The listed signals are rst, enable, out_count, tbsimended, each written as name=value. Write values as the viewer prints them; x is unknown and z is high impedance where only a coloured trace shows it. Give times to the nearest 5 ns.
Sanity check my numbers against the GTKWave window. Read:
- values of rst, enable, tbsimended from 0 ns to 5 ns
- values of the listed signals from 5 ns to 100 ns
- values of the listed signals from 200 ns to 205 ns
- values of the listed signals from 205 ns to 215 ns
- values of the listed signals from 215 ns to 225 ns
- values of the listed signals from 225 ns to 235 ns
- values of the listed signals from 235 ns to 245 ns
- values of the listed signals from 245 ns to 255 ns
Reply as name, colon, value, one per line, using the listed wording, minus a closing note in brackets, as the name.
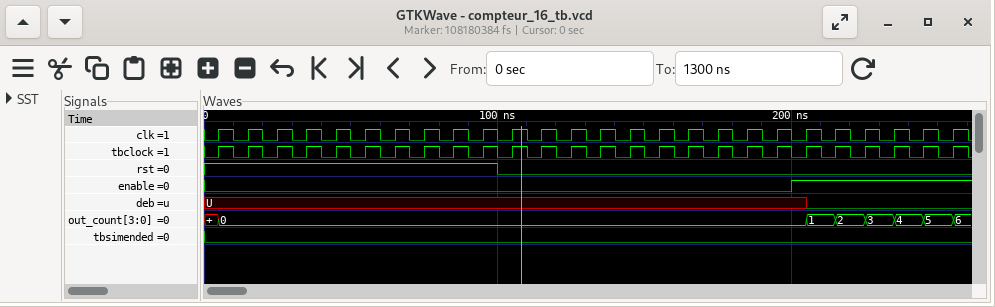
values of rst, enable, tbsimended from 0 ns to 5 ns: rst=1, enable=0, tbsimended=0
values of the listed signals from 5 ns to 100 ns: rst=1, enable=0, out_count=0, tbsimended=0
values of the listed signals from 200 ns to 205 ns: rst=0, enable=1, out_count=0, tbsimended=0
values of the listed signals from 205 ns to 215 ns: rst=0, enable=1, out_count=1, tbsimended=0
values of the listed signals from 215 ns to 225 ns: rst=0, enable=1, out_count=2, tbsimended=0
values of the listed signals from 225 ns to 235 ns: rst=0, enable=1, out_count=3, tbsimended=0
values of the listed signals from 235 ns to 245 ns: rst=0, enable=1, out_count=4, tbsimended=0
values of the listed signals from 245 ns to 255 ns: rst=0, enable=1, out_count=5, tbsimended=0
